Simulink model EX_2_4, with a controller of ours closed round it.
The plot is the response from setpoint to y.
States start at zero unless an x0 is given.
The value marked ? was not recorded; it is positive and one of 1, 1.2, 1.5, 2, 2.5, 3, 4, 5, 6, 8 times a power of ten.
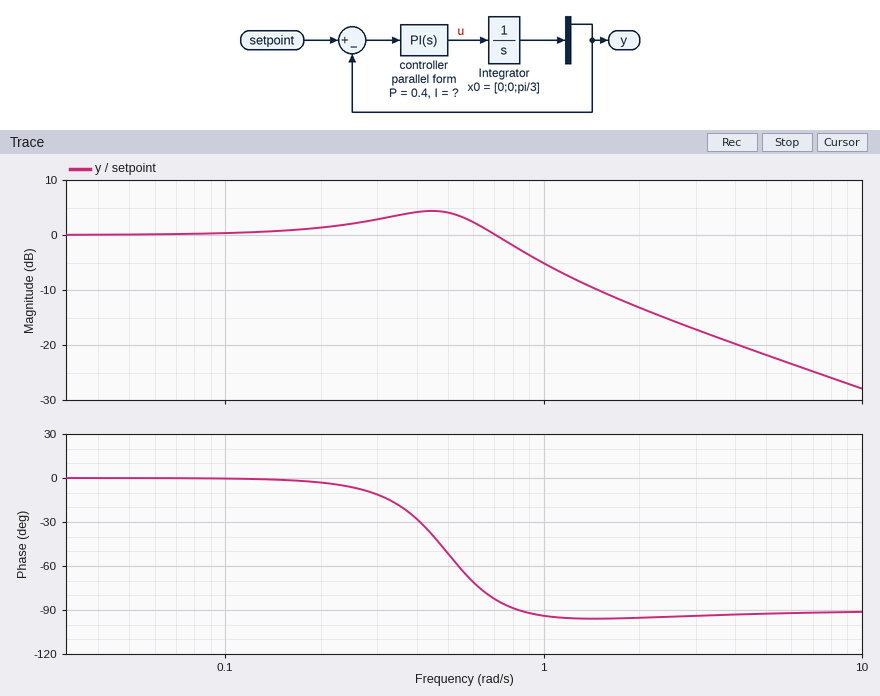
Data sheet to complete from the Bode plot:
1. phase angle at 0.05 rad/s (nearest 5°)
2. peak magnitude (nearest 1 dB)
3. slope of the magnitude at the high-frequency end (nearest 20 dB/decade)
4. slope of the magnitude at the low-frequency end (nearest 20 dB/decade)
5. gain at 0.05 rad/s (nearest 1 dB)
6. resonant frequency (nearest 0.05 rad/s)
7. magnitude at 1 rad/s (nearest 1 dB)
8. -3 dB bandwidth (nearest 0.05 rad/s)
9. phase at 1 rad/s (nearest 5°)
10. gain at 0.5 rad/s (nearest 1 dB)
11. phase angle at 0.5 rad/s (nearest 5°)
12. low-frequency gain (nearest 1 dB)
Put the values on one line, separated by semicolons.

0°; 4 dB; -20 dB/decade; 0 dB/decade; 0 dB; 0.45 rad/s; -5 dB; 0.85 rad/s; -95°; 4 dB; -50°; 0 dB
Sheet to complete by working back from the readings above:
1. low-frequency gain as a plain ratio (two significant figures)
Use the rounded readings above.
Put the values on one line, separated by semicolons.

1.0
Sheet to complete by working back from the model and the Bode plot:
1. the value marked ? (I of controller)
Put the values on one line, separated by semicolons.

0.25
